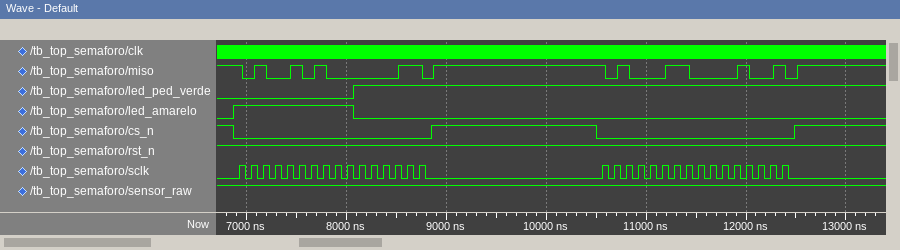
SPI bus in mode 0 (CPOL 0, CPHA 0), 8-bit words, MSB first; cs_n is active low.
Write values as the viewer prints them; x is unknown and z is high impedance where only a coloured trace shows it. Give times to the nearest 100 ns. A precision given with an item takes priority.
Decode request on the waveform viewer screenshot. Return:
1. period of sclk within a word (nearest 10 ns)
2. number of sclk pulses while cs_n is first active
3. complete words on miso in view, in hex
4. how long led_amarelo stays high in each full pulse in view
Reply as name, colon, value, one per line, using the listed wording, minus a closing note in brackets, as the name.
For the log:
period of sclk within a word: 120 ns
number of sclk pulses while cs_n is first active: 16
complete words on miso in view, in hex: A5, 03, A3, 09
how long led_amarelo stays high in each full pulse in view: 1200 ns
